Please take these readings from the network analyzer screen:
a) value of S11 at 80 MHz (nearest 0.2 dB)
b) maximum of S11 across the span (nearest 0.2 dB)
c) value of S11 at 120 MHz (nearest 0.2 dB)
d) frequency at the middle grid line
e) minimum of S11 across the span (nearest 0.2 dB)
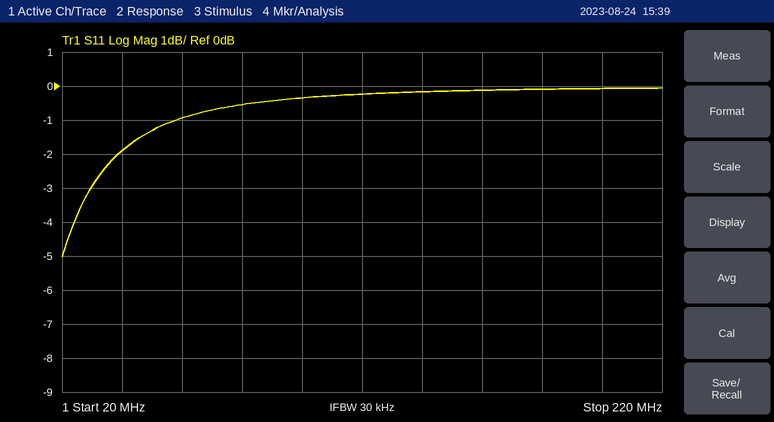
-0.6 dB
0.0 dB
-0.2 dB
120 MHz
-5.0 dB
